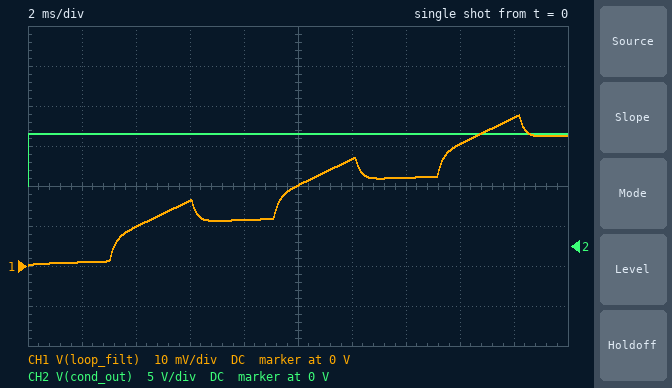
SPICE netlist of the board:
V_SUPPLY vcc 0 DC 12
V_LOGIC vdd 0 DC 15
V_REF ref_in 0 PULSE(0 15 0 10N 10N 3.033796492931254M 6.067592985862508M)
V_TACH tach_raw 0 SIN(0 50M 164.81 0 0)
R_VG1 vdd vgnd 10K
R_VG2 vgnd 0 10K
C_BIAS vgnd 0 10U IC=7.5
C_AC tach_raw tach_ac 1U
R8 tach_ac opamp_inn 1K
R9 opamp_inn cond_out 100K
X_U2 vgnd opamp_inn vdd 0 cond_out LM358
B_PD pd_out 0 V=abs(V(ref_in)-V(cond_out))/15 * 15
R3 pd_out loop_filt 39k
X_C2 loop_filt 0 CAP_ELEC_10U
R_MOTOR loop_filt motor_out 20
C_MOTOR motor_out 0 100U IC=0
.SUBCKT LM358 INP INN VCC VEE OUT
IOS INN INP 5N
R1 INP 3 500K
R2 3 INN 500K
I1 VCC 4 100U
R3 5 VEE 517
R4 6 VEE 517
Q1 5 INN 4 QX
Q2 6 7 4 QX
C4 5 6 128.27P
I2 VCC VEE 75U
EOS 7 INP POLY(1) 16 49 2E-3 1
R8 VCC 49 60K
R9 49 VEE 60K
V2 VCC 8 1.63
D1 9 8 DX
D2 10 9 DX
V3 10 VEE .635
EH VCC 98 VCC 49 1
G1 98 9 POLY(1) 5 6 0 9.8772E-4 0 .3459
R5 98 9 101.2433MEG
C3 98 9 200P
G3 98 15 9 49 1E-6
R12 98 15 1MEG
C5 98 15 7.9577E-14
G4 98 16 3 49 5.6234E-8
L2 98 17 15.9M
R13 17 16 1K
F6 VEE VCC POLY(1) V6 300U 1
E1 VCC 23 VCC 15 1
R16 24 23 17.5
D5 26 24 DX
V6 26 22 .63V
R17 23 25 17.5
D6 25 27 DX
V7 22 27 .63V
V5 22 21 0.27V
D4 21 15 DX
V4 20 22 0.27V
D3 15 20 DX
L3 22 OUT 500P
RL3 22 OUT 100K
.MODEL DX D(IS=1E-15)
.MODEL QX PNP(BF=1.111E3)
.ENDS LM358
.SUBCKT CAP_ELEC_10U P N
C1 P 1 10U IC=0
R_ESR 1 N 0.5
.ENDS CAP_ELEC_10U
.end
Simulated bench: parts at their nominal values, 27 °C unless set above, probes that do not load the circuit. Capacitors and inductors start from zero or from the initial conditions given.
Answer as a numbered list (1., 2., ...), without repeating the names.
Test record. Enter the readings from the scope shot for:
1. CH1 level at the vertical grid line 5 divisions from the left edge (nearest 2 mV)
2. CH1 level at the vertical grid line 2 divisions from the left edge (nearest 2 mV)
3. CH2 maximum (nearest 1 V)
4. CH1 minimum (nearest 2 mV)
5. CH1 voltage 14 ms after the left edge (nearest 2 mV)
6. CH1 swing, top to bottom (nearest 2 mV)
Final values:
1. 20 mV
2. 10 mV
3. 14 V
4. 0 V
5. 22 mV
6. 38 mV
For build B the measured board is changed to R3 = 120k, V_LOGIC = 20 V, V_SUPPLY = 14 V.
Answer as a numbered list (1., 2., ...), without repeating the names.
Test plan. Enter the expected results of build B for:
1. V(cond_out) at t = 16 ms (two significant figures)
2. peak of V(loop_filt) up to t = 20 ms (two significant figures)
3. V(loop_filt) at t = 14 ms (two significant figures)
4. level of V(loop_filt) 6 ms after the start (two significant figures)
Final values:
1. 19 V
2. 18 mV
3. 12 mV
4. 7.8 mV
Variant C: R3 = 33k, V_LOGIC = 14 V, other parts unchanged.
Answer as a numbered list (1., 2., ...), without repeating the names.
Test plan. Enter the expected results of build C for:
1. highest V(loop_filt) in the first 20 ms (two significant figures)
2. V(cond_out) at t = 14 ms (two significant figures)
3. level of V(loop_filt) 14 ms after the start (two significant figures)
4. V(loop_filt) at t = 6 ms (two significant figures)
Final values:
1. 44 mV
2. 13 V
3. 27 mV
4. 19 mV
